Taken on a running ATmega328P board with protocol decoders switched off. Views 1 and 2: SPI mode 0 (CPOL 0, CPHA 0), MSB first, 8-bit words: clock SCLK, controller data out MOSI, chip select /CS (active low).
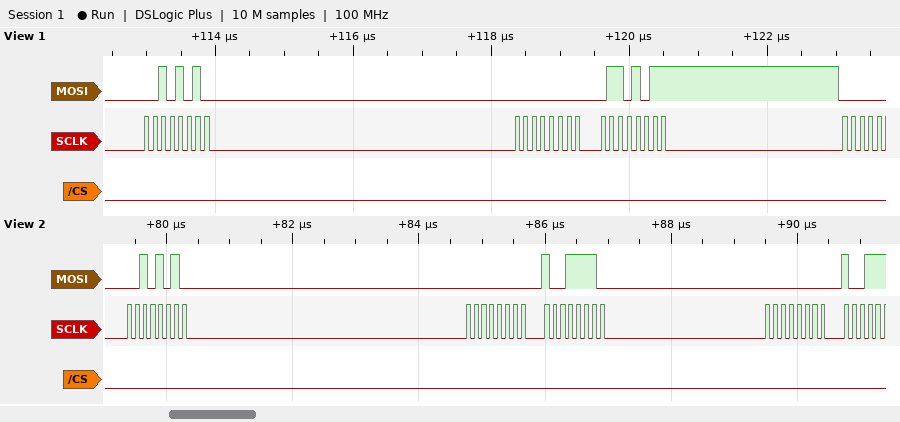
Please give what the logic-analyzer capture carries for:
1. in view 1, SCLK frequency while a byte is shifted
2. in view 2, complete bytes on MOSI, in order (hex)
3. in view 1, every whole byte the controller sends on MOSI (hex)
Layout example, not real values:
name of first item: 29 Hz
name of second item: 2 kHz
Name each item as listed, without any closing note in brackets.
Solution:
in view 1, SCLK frequency while a byte is shifted: 8 MHz
in view 2, complete bytes on MOSI, in order: 2A 00 9E 00
in view 1, every whole byte the controller sends on MOSI: 2A 00 6B
